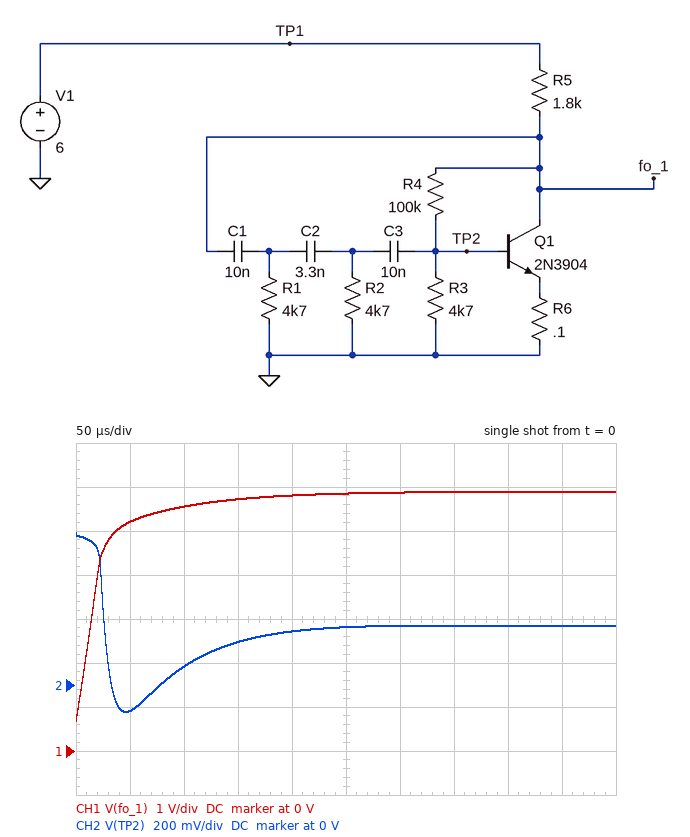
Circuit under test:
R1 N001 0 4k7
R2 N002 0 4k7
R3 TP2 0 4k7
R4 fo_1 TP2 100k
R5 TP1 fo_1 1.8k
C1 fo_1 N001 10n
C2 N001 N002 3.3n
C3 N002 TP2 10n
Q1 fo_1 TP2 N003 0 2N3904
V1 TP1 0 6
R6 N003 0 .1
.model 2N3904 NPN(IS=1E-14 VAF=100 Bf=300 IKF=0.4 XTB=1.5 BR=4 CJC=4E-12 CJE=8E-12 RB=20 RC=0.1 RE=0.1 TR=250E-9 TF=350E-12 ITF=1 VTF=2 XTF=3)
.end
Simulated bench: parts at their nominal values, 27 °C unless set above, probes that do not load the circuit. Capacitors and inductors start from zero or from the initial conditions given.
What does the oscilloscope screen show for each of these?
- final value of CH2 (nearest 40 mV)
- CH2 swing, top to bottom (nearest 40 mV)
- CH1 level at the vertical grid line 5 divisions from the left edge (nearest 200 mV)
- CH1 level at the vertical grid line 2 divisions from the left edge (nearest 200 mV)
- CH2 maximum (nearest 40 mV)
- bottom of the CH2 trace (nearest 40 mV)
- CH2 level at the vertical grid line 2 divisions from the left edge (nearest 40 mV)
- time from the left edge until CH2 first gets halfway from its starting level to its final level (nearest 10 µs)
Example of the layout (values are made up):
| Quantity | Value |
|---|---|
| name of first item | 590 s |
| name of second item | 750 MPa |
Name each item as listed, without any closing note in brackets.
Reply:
| Quantity | Value |
|---|---|
| final value of CH2 | 280 mV |
| CH2 swing, top to bottom | 800 mV |
| CH1 level at the vertical grid line 5 divisions from the left edge | 5.8 V |
| CH1 level at the vertical grid line 2 divisions from the left edge | 5.6 V |
| CH2 maximum | 680 mV |
| bottom of the CH2 trace | -120 mV |
| CH2 level at the vertical grid line 2 divisions from the left edge | 80 mV |
| time from the left edge until CH2 first gets halfway from its starting level to its final level | 20 µs |
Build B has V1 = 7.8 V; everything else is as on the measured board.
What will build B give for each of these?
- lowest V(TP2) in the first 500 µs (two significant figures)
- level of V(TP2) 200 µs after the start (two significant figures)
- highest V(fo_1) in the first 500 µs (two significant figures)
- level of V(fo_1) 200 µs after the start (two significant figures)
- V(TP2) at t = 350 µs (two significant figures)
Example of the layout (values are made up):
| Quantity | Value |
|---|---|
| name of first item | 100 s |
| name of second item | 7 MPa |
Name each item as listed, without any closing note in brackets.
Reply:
| Quantity | Value |
|---|---|
| lowest V(TP2) in the first 500 µs | -150 mV |
| level of V(TP2) 200 µs after the start | 310 mV |
| highest V(fo_1) in the first 500 µs | 7.7 V |
| level of V(fo_1) 200 µs after the start | 7.5 V |
| V(TP2) at t = 350 µs | 350 mV |
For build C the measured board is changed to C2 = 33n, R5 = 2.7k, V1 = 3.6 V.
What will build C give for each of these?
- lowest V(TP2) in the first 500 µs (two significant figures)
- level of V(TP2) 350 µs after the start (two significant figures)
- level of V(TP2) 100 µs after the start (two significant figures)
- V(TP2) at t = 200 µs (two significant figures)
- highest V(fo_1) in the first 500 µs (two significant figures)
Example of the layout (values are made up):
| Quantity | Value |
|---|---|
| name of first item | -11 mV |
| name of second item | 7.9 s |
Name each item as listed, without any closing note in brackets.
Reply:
| Quantity | Value |
|---|---|
| lowest V(TP2) in the first 500 µs | -66 mV |
| level of V(TP2) 350 µs after the start | 150 mV |
| level of V(TP2) 100 µs after the start | -60 mV |
| V(TP2) at t = 200 µs | 80 mV |
| highest V(fo_1) in the first 500 µs | 3.5 V |
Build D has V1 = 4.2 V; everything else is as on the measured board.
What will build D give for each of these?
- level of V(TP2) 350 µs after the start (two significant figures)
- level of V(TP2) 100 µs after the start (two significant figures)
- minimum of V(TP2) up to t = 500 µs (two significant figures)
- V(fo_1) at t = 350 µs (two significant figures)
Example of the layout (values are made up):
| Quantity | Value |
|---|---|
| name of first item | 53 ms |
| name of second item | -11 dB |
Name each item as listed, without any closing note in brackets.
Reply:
| Quantity | Value |
|---|---|
| level of V(TP2) 350 µs after the start | 190 mV |
| level of V(TP2) 100 µs after the start | 67 mV |
| minimum of V(TP2) up to t = 500 µs | -93 mV |
| V(fo_1) at t = 350 µs | 4.1 V |
